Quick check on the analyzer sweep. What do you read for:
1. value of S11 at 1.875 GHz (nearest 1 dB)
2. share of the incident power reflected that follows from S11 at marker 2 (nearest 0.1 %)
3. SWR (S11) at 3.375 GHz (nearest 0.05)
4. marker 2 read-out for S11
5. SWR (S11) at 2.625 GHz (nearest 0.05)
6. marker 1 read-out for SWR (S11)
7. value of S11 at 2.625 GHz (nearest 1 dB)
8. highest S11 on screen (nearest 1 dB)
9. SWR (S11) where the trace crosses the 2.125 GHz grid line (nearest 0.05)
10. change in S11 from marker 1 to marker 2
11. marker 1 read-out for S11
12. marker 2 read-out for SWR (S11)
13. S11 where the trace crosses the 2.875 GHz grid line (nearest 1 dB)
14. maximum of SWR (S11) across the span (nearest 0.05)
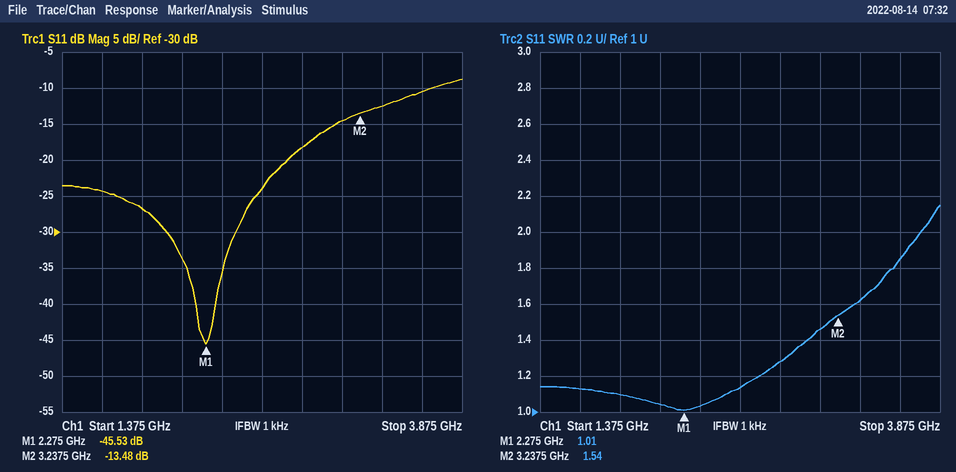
-27 dB
4.5 %
1.60
-13.48 dB
1.15
1.01
-24 dB
-9 dB
1.05
32.05 dB
-45.53 dB
1.54
-18 dB
2.15
